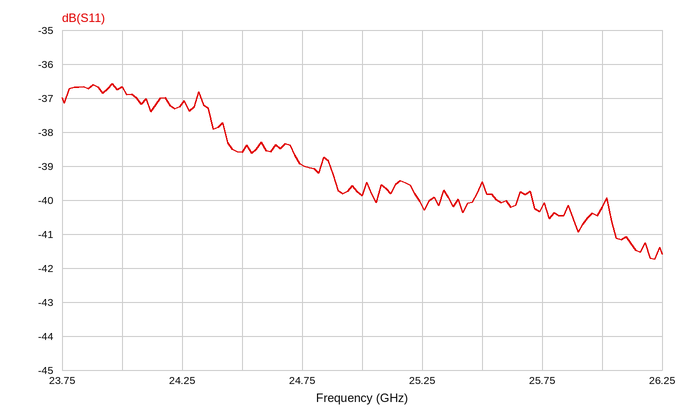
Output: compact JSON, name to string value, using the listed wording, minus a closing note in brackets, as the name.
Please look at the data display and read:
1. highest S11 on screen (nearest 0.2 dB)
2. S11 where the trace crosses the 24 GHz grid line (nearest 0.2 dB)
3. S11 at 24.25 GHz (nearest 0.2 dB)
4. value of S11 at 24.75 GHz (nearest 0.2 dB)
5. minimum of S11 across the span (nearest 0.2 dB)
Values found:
{"highest S11 on screen": "-36.6 dB", "S11 where the trace crosses the 24 GHz grid line": "-36.6 dB", "S11 at 24.25 GHz": "-37.2 dB", "value of S11 at 24.75 GHz": "-39.0 dB", "minimum of S11 across the span": "-41.8 dB"}
